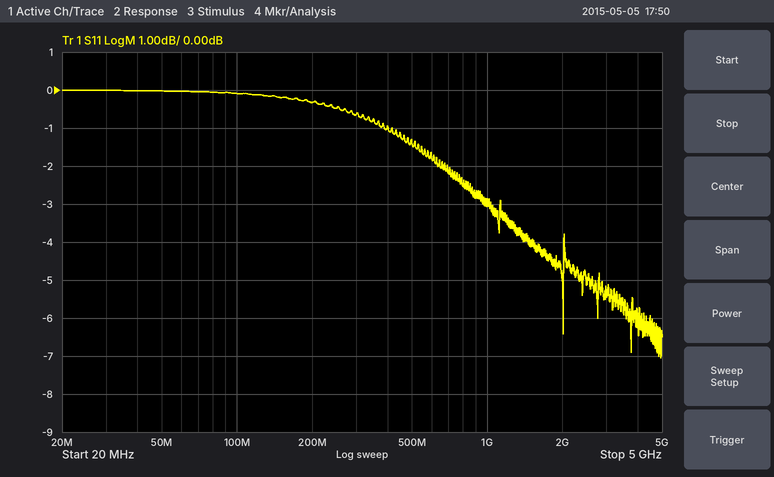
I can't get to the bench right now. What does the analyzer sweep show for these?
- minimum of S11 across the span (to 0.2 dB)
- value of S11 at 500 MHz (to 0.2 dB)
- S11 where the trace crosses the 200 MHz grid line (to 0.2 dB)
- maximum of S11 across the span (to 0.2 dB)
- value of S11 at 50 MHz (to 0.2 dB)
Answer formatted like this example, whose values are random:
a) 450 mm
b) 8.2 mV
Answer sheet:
a) -7.0 dB
b) -1.4 dB
c) -0.4 dB
d) 0.0 dB
e) 0.0 dB
